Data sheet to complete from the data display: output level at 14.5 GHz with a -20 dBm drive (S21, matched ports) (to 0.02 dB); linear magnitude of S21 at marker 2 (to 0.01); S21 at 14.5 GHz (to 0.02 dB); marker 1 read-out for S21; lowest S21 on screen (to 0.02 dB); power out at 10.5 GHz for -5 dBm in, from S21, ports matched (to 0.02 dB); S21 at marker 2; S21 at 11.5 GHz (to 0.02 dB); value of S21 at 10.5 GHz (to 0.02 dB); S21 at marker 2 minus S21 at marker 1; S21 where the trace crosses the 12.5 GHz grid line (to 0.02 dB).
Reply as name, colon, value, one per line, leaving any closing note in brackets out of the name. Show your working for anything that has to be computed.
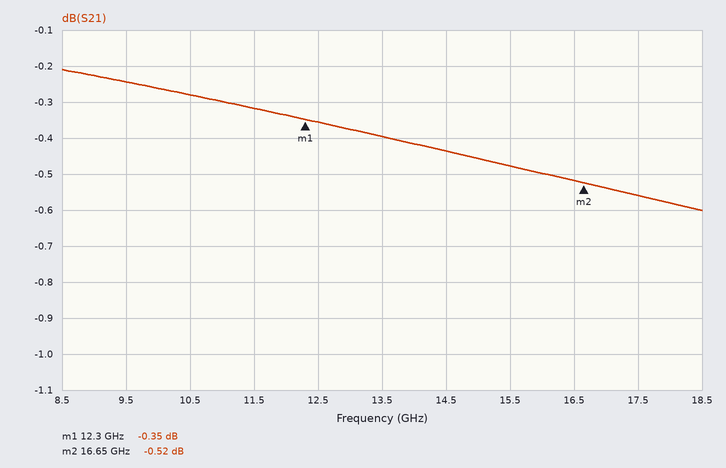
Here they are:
output level at 14.5 GHz with a -20 dBm drive (S21, matched ports): -20 dBm + (-0.44 dB) = -20.44 dBm
linear magnitude of S21 at marker 2: 10^(-0.52/20) ≈ 0.94
S21 at 14.5 GHz: -0.44 dB
marker 1 read-out for S21: -0.35 dB
lowest S21 on screen: -0.60 dB
power out at 10.5 GHz for -5 dBm in, from S21, ports matched: -5 dBm + (-0.28 dB) = -5.28 dBm
S21 at marker 2: -0.52 dB
S21 at 11.5 GHz: -0.32 dB
value of S21 at 10.5 GHz: -0.28 dB
S21 at marker 2 minus S21 at marker 1: -0.52 − (-0.35) = -0.17 dB
S21 where the trace crosses the 12.5 GHz grid line: -0.36 dB
